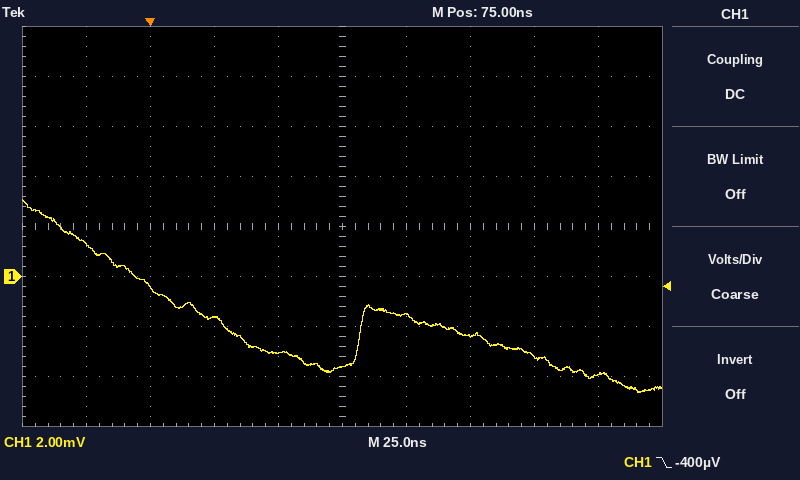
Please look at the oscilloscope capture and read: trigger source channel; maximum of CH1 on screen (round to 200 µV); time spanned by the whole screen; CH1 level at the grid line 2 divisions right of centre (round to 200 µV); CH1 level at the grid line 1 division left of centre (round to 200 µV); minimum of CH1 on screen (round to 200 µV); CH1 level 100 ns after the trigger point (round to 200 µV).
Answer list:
CH1
3.0 mV
250 ns
-2.4 mV
-3.0 mV
-4.6 mV
-1.6 mV
